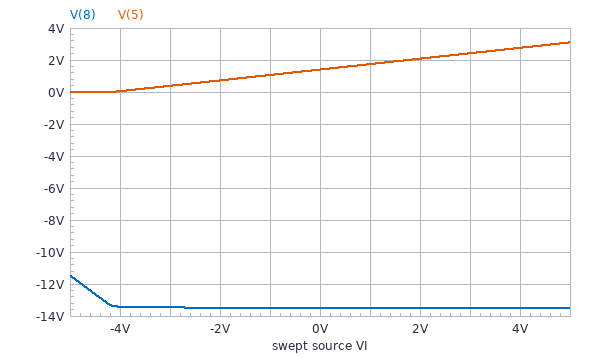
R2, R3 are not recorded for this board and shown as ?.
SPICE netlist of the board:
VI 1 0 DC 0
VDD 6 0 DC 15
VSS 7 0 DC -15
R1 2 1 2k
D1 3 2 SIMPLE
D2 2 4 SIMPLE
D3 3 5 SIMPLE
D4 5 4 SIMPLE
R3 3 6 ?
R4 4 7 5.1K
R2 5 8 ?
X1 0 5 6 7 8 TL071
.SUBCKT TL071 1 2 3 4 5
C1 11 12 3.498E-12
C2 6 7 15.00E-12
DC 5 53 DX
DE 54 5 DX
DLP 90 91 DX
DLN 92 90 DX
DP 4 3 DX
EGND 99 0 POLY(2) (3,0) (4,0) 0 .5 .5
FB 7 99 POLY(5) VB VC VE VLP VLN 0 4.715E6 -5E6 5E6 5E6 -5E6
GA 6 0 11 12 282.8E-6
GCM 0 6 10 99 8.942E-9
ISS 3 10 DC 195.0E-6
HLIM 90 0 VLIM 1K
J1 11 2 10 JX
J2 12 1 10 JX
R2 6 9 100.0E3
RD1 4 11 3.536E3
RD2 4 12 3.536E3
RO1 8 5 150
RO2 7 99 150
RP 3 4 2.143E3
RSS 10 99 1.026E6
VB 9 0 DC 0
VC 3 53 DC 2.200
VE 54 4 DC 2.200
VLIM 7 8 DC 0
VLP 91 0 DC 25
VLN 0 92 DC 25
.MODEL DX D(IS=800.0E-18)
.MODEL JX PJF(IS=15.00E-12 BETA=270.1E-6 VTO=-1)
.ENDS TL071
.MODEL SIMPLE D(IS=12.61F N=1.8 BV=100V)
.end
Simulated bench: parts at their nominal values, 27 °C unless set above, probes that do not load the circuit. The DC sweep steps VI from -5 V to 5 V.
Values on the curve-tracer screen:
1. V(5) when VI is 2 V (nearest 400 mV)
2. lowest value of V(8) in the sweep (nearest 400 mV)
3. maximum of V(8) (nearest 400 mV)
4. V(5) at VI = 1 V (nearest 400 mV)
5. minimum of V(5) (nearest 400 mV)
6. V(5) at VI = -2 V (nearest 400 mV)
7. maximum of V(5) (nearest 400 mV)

2.0 V
-13.6 V
-11.6 V
1.6 V
0 V
800 mV
3.2 V
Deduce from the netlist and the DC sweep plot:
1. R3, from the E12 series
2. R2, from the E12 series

1.8 kΩ
4.7 kΩ
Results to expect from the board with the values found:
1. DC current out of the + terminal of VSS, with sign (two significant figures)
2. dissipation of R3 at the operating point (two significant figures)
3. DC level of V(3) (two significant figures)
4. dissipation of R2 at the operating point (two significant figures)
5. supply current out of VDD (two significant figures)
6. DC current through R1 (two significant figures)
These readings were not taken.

-17 mA
85 mW
2.6 V
47 mW
21 mA
710 µA
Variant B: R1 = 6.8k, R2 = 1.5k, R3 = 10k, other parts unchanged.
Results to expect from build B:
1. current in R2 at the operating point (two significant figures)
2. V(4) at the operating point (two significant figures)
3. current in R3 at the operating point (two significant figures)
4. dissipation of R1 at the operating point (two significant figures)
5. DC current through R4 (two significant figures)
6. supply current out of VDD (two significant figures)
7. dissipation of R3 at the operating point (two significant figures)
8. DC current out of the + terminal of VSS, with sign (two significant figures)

1.3 mA
-1.2 V
1.4 mA
140 nW
2.7 mA
16 mA
19 mW
-17 mA
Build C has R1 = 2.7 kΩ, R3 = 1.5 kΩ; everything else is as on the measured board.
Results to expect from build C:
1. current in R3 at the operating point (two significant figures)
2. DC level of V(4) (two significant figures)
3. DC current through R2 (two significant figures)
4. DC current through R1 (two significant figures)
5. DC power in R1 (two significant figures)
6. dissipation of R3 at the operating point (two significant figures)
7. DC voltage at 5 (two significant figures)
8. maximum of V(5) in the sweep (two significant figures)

7.5 mA
1.3 V
3.4 mA
930 µA
2.3 mW
85 mW
2.5 V
3.8 V
